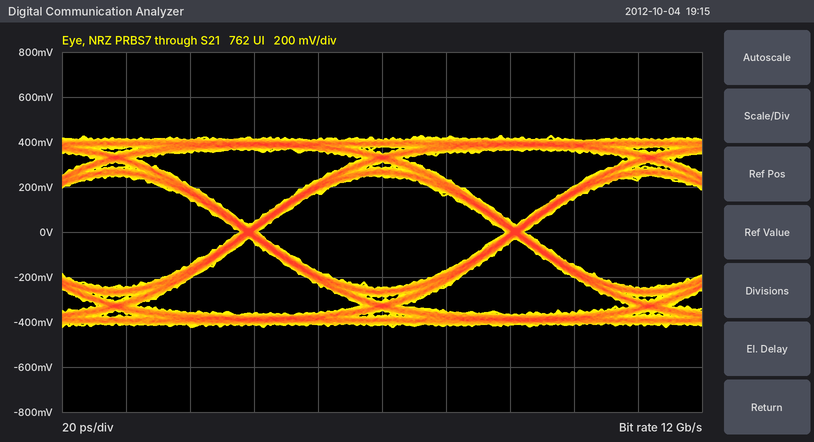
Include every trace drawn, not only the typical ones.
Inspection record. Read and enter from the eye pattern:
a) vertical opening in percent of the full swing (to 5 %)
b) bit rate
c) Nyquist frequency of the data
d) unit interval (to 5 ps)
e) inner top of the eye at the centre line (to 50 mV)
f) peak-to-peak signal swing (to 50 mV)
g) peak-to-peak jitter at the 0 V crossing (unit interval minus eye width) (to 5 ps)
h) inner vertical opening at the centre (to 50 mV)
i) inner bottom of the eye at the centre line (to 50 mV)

60 %
12 Gb/s
6 GHz
85 ps
250 mV
850 mV
5 ps
500 mV
-250 mV
